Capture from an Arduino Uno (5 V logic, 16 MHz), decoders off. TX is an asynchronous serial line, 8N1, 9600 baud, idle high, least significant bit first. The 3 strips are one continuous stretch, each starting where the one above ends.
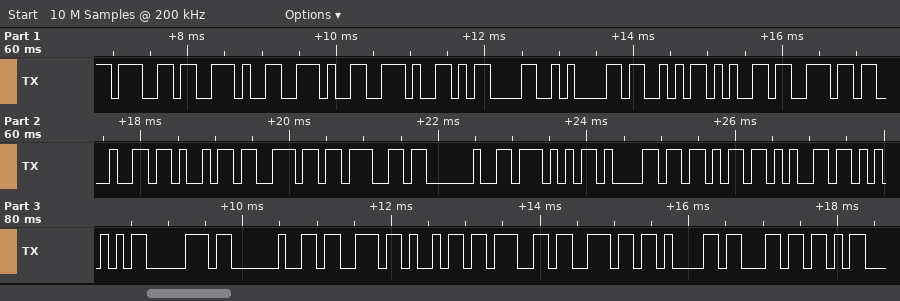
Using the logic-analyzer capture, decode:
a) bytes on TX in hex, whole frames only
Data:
67 2E 2E 2E 0D 0A 53 65 6E 64 69 6E 67 20 57 61 6B 65 55 70 20 73 69 67 6E 61 6C
